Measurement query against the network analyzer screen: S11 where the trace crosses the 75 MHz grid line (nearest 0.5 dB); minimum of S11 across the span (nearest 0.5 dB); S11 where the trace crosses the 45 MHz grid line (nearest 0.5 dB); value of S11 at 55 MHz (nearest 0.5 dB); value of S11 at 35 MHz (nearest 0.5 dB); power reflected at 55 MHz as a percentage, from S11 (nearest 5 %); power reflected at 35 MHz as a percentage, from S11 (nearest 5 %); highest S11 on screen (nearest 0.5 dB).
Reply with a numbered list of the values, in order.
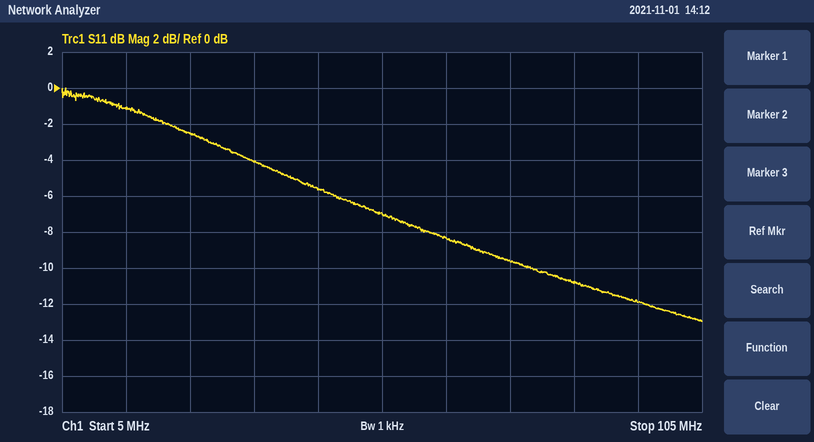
1. -9.5 dB
2. -13.0 dB
3. -5.5 dB
4. -7.0 dB
5. -4.0 dB
6. 20 %
7. 40 %
8. 0.0 dB
